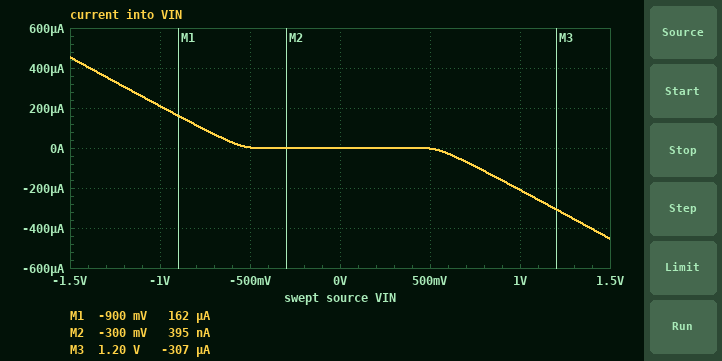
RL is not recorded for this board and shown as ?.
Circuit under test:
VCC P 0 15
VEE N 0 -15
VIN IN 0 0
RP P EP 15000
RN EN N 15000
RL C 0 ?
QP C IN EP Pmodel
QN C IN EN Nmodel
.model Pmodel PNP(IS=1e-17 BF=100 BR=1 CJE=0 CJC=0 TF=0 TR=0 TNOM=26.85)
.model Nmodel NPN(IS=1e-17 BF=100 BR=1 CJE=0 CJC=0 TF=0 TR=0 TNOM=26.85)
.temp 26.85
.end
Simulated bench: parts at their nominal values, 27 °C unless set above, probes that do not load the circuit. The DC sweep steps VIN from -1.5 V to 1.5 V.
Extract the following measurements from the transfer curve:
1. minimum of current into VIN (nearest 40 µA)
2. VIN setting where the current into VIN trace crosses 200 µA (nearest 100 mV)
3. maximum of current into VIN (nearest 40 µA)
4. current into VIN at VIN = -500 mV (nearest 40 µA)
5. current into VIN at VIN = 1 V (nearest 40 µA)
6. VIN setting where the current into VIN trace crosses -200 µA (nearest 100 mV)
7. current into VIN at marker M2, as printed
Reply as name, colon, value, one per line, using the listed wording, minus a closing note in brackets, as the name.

minimum of current into VIN: -440 µA
VIN setting where the current into VIN trace crosses 200 µA: -1.0 V
maximum of current into VIN: 440 µA
current into VIN at VIN = -500 mV: 0 A
current into VIN at VIN = 1 V: -200 µA
VIN setting where the current into VIN trace crosses -200 µA: 1.0 V
current into VIN at marker M2, as printed: 395 nA
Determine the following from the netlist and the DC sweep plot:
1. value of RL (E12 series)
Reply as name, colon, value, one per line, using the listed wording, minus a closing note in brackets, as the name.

value of RL: 2.7 kΩ
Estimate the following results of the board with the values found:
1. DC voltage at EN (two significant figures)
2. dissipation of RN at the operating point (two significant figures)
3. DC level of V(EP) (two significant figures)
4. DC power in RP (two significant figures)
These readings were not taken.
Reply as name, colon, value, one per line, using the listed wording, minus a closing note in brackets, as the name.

DC voltage at EN: -830 mV
dissipation of RN at the operating point: 13 mW
DC level of V(EP): 830 mV
DC power in RP: 13 mW
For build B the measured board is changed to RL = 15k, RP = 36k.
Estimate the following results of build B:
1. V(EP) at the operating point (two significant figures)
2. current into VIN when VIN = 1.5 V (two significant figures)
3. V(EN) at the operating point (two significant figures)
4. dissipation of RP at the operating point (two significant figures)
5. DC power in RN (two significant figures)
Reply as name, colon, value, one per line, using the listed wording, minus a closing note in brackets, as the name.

V(EP) at the operating point: 810 mV
current into VIN when VIN = 1.5 V: -740 µA
V(EN) at the operating point: -840 mV
dissipation of RP at the operating point: 5.6 mW
DC power in RN: 13 mW
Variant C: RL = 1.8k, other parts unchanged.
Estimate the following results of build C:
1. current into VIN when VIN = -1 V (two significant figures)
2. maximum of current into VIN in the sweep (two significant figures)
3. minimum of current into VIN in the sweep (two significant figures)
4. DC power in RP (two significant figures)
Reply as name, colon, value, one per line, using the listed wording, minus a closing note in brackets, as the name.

current into VIN when VIN = -1 V: 250 µA
maximum of current into VIN in the sweep: 580 µA
minimum of current into VIN in the sweep: -580 µA
DC power in RP: 13 mW
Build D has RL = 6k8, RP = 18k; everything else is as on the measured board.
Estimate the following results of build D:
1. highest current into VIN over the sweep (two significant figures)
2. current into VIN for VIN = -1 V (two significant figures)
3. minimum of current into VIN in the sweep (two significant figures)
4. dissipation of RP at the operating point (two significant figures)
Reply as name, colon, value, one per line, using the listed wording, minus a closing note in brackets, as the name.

highest current into VIN over the sweep: 130 µA
current into VIN for VIN = -1 V: 7.7 µA
minimum of current into VIN in the sweep: -440 µA
dissipation of RP at the operating point: 11 mW
